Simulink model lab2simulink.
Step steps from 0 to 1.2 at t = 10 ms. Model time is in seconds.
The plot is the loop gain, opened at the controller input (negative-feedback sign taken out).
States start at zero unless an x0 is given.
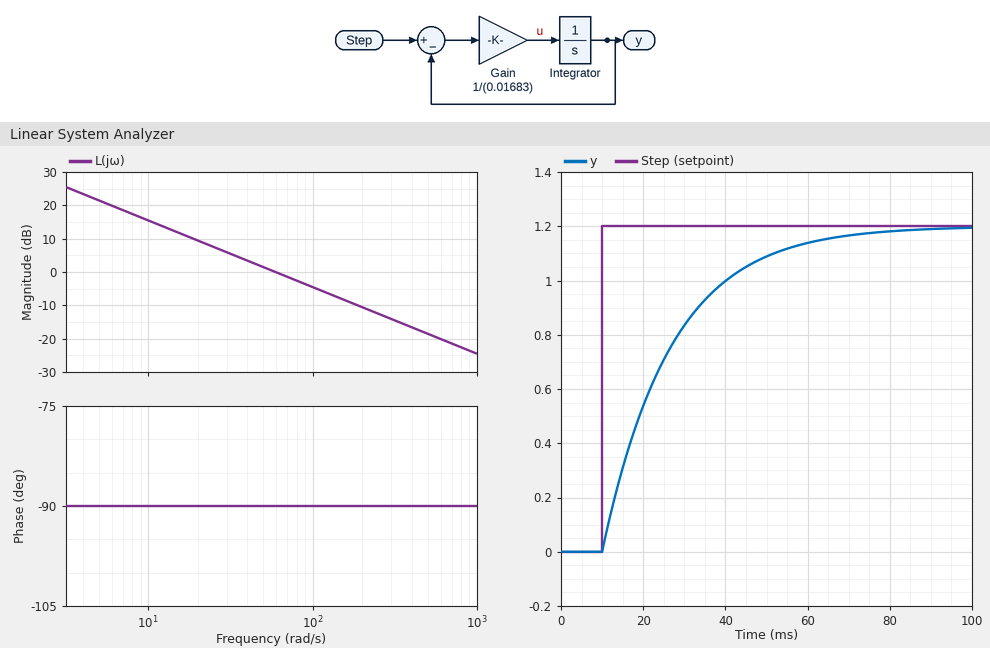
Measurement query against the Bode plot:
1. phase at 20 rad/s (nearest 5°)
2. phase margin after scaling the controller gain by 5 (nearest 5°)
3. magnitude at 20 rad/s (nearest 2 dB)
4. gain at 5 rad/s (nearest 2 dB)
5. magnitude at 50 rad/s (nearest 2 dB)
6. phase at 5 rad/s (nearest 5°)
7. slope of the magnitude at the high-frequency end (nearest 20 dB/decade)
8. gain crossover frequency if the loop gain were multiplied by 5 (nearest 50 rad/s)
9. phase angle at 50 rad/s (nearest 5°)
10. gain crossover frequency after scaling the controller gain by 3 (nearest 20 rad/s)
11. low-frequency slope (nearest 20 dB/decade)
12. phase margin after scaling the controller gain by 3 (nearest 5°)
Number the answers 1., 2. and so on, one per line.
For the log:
1. -90°
2. 90°
3. 10 dB
4. 22 dB
5. 2 dB
6. -90°
7. -20 dB/decade
8. 300 rad/s
9. -90°
10. 180 rad/s
11. -20 dB/decade
12. 90°
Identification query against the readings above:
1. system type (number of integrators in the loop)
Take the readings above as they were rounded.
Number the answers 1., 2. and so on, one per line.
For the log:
1. 1
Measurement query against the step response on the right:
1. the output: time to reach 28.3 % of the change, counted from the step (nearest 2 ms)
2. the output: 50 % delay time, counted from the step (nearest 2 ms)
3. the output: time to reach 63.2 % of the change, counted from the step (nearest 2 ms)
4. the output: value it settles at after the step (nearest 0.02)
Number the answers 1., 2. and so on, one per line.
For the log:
1. 6 ms
2. 12 ms
3. 16 ms
4. 1.20
